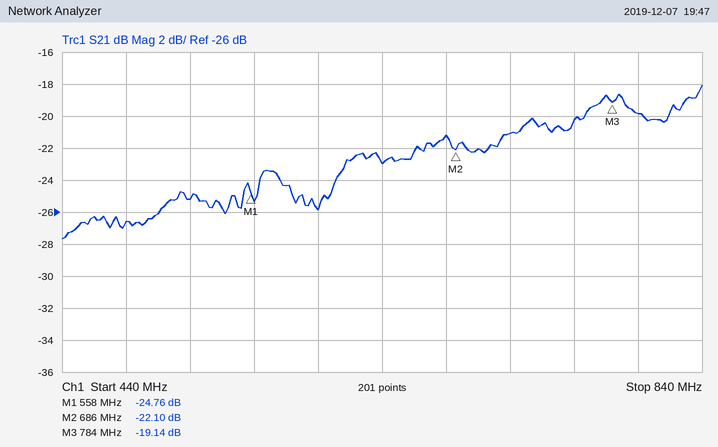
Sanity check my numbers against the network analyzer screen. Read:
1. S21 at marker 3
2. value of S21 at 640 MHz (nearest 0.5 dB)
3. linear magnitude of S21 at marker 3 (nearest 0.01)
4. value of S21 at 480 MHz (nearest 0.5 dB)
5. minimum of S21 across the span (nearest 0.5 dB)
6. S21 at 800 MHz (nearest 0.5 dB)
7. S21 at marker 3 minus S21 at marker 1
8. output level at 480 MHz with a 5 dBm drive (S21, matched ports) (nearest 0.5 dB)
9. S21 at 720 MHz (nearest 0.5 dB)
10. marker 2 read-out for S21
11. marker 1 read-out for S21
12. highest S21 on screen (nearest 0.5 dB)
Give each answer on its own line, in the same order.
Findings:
-19.14 dB
-23.0 dB
0.11
-26.5 dB
-27.5 dB
-20.0 dB
5.62 dB
-21.5 dBm
-21.0 dB
-22.10 dB
-24.76 dB
-18.0 dB
